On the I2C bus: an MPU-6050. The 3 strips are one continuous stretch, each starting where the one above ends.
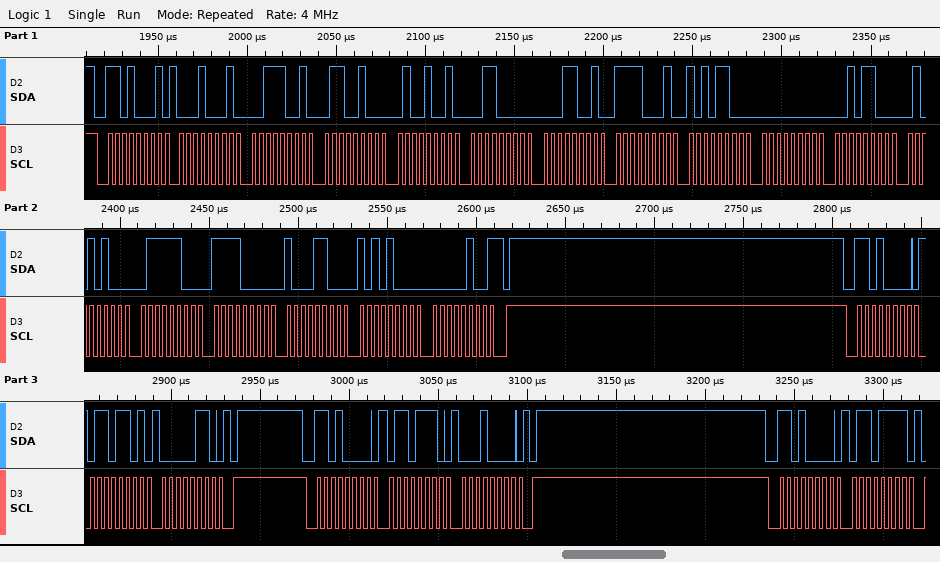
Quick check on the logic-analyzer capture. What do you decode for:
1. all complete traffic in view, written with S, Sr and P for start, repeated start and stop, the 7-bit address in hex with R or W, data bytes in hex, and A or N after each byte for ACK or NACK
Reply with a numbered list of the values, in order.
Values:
1. S 68R A 11 A 39 A 64 A 49 A 30 A 19 A F1 A AC A 00 A 2C A 54 A 7C A F0 A 8C A A8 A 04 N P S 68W A 6D A 06 A P S 68W A 6E A 10 A P S 68W A 6F A
